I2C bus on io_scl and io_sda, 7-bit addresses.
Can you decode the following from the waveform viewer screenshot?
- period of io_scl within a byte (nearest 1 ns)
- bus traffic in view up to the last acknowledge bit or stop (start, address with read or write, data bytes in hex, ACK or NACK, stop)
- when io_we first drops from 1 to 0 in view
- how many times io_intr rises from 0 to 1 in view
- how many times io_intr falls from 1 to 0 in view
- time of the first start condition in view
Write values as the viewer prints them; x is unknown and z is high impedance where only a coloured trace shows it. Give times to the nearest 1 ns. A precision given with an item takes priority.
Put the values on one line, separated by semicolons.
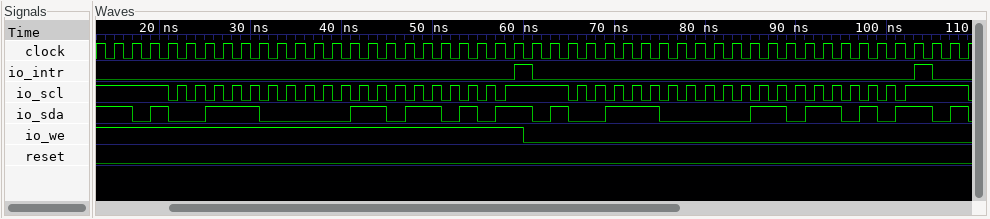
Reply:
2 ns; start, address 1C write ACK, 6D ACK, repeated start, address 1C write ACK, 6D ACK; 60 ns; 2; 2; 17 ns
